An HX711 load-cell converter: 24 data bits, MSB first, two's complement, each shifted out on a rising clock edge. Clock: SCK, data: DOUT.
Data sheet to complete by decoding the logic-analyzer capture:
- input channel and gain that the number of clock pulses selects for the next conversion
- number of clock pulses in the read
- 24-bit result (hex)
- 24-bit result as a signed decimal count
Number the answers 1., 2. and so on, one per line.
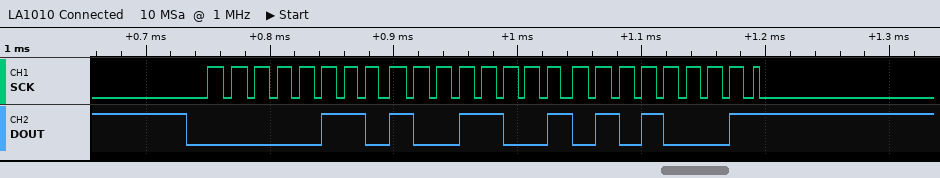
1. channel A, gain 128
2. 25
3. 0x069951
4. 432465
